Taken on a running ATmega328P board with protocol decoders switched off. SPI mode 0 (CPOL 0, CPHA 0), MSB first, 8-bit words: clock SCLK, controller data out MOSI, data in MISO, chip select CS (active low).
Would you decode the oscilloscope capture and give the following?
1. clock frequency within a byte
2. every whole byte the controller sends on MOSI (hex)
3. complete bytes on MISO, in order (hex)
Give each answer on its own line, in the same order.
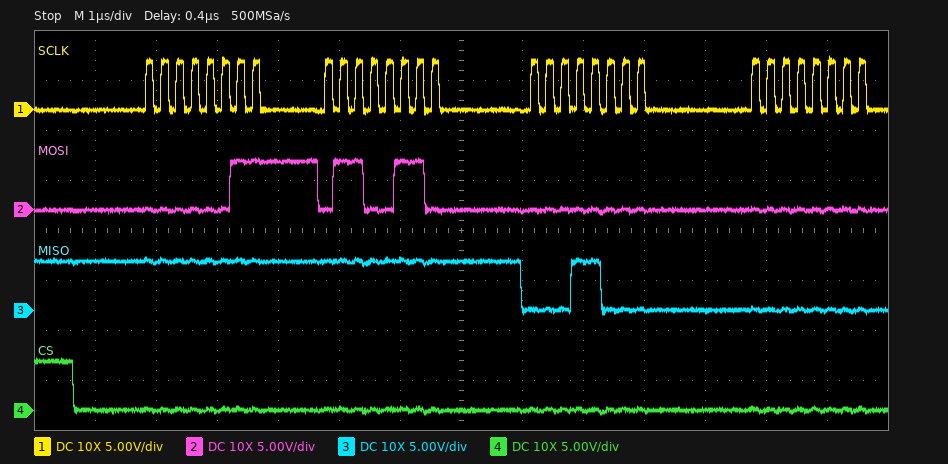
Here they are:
4 MHz
03 66 00 00
FF FF 18 00
